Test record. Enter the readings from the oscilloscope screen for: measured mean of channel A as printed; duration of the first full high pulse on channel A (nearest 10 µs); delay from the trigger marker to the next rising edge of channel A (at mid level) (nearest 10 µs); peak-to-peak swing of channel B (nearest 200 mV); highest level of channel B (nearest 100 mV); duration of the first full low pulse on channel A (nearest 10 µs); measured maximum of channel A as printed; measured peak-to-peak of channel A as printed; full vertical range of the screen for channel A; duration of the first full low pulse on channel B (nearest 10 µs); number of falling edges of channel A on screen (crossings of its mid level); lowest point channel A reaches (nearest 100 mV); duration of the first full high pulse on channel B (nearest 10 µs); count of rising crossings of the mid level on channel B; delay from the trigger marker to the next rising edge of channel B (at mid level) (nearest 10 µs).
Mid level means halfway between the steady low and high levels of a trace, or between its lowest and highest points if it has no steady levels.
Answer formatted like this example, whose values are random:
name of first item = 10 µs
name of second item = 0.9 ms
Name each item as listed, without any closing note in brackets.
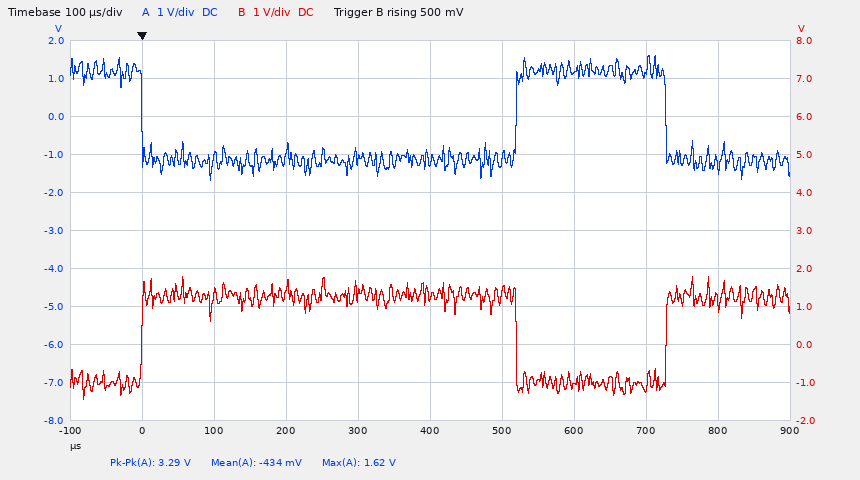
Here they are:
measured mean of channel A as printed = -434 mV
duration of the first full high pulse on channel A = 210 µs
delay from the trigger marker to the next rising edge of channel A (at mid level) = 520 µs
peak-to-peak swing of channel B = 3.2 V
highest level of channel B = 1.8 V
duration of the first full low pulse on channel A = 520 µs
measured maximum of channel A as printed = 1.62 V
measured peak-to-peak of channel A as printed = 3.29 V
full vertical range of the screen for channel A = 10 V
duration of the first full low pulse on channel B = 210 µs
number of falling edges of channel A on screen = 2
lowest point channel A reaches = -1.7 V
duration of the first full high pulse on channel B = 520 µs
count of rising crossings of the mid level on channel B = 2
delay from the trigger marker to the next rising edge of channel B (at mid level) = 730 µs
